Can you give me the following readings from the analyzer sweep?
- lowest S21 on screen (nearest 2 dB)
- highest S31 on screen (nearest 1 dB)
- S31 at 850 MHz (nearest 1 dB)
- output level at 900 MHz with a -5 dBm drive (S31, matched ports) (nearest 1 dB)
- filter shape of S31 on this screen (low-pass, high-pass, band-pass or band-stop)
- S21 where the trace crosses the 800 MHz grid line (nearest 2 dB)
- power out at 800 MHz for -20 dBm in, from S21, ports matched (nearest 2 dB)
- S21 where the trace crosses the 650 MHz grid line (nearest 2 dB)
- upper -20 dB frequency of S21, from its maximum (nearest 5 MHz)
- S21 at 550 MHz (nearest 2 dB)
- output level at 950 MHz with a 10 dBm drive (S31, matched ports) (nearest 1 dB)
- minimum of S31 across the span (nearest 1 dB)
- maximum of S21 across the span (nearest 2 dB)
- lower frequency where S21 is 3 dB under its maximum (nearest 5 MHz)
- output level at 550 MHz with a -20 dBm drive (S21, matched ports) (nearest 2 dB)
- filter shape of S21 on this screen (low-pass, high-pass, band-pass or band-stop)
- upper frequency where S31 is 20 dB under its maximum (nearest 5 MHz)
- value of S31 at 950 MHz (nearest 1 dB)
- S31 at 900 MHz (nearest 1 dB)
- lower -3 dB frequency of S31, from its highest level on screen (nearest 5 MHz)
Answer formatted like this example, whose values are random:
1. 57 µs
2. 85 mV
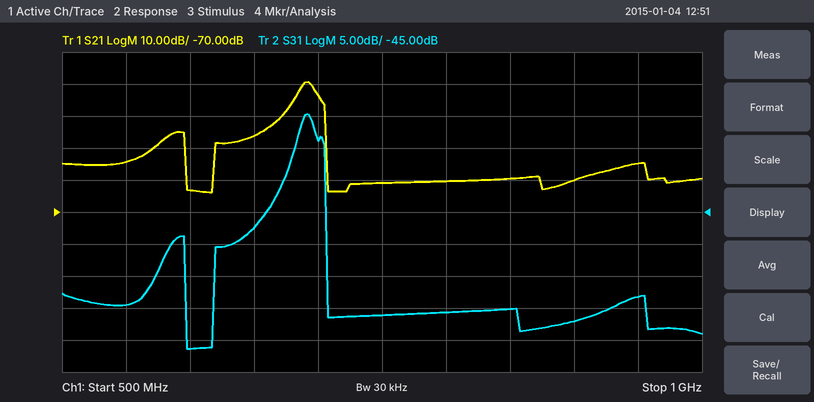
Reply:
1. -64 dB
2. -30 dB
3. -60 dB
4. -67 dBm
5. band-pass
6. -60 dB
7. -80 dBm
8. -46 dB
9. 705 MHz
10. -54 dB
11. -48 dBm
12. -66 dB
13. -30 dB
14. 685 MHz
15. -74 dBm
16. band-pass
17. 705 MHz
18. -58 dB
19. -62 dB
20. 685 MHz
